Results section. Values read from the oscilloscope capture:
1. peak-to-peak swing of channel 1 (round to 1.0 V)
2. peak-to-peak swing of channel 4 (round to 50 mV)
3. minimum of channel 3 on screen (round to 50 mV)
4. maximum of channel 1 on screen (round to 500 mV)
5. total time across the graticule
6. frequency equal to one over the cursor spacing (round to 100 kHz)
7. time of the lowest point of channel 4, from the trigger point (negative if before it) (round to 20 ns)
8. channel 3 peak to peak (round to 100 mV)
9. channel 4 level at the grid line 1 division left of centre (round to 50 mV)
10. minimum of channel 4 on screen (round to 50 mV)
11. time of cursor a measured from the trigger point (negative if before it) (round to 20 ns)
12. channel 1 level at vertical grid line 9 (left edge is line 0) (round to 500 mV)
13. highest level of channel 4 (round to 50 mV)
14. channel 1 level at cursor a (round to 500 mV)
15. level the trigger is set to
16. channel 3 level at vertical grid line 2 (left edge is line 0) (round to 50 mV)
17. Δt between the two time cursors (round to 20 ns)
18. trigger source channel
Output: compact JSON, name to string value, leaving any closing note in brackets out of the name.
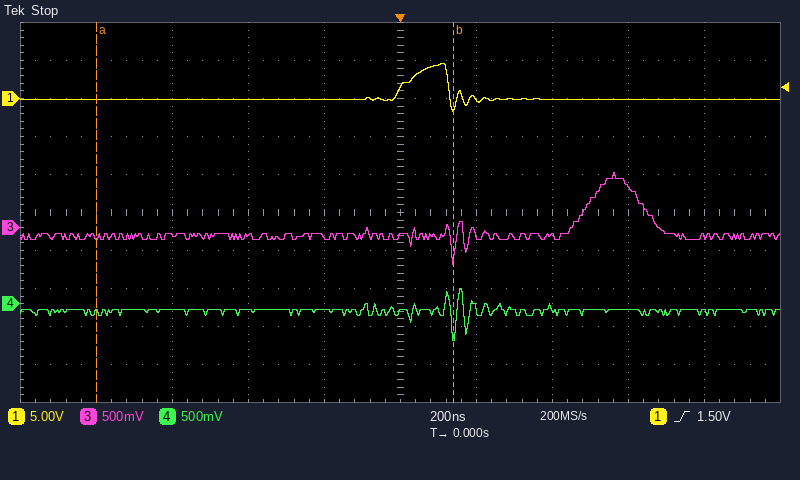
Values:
{"peak-to-peak swing of channel 1": "6.0 V", "peak-to-peak swing of channel 4": "700 mV", "minimum of channel 3 on screen": "-500 mV", "maximum of channel 1 on screen": "4.5 V", "total time across the graticule": "2 µs", "frequency equal to one over the cursor spacing": "1.1 MHz", "time of the lowest point of channel 4, from the trigger point (negative if before it)": "+140 ns", "channel 3 peak to peak": "1.20 V", "channel 4 level at the grid line 1 division left of centre": "-100 mV", "minimum of channel 4 on screen": "-500 mV", "time of cursor a measured from the trigger point (negative if before it)": "-800 ns", "channel 1 level at vertical grid line 9 (left edge is line 0)": "0.0 V", "highest level of channel 4": "200 mV", "channel 1 level at cursor a": "0.0 V", "level the trigger is set to": "1.50 V", "channel 3 level at vertical grid line 2 (left edge is line 0)": "-100 mV", "Δt between the two time cursors": "940 ns", "trigger source channel": "channel 1"}
